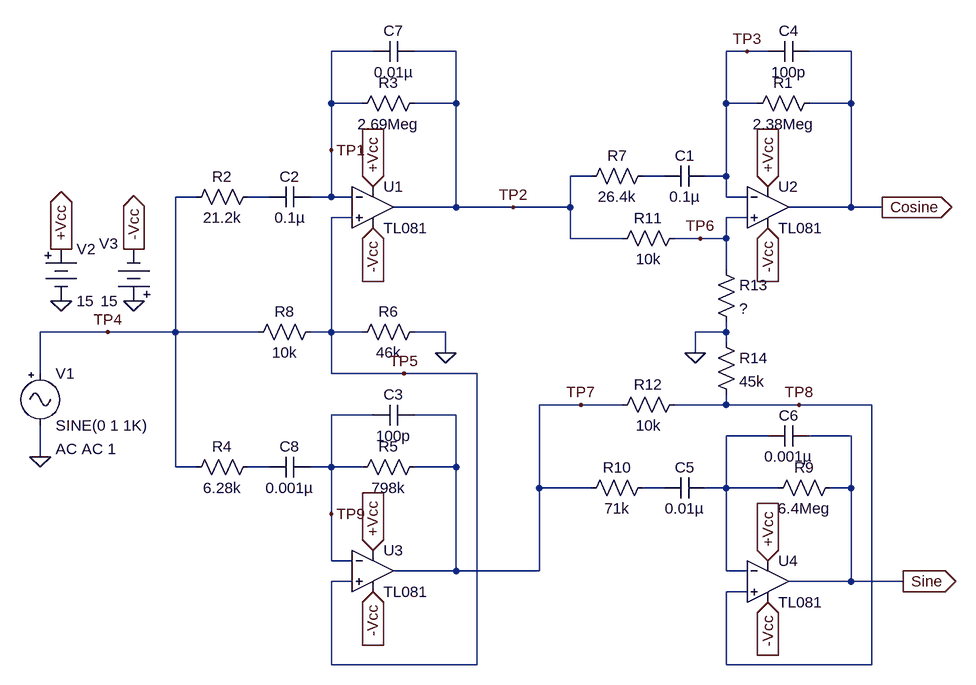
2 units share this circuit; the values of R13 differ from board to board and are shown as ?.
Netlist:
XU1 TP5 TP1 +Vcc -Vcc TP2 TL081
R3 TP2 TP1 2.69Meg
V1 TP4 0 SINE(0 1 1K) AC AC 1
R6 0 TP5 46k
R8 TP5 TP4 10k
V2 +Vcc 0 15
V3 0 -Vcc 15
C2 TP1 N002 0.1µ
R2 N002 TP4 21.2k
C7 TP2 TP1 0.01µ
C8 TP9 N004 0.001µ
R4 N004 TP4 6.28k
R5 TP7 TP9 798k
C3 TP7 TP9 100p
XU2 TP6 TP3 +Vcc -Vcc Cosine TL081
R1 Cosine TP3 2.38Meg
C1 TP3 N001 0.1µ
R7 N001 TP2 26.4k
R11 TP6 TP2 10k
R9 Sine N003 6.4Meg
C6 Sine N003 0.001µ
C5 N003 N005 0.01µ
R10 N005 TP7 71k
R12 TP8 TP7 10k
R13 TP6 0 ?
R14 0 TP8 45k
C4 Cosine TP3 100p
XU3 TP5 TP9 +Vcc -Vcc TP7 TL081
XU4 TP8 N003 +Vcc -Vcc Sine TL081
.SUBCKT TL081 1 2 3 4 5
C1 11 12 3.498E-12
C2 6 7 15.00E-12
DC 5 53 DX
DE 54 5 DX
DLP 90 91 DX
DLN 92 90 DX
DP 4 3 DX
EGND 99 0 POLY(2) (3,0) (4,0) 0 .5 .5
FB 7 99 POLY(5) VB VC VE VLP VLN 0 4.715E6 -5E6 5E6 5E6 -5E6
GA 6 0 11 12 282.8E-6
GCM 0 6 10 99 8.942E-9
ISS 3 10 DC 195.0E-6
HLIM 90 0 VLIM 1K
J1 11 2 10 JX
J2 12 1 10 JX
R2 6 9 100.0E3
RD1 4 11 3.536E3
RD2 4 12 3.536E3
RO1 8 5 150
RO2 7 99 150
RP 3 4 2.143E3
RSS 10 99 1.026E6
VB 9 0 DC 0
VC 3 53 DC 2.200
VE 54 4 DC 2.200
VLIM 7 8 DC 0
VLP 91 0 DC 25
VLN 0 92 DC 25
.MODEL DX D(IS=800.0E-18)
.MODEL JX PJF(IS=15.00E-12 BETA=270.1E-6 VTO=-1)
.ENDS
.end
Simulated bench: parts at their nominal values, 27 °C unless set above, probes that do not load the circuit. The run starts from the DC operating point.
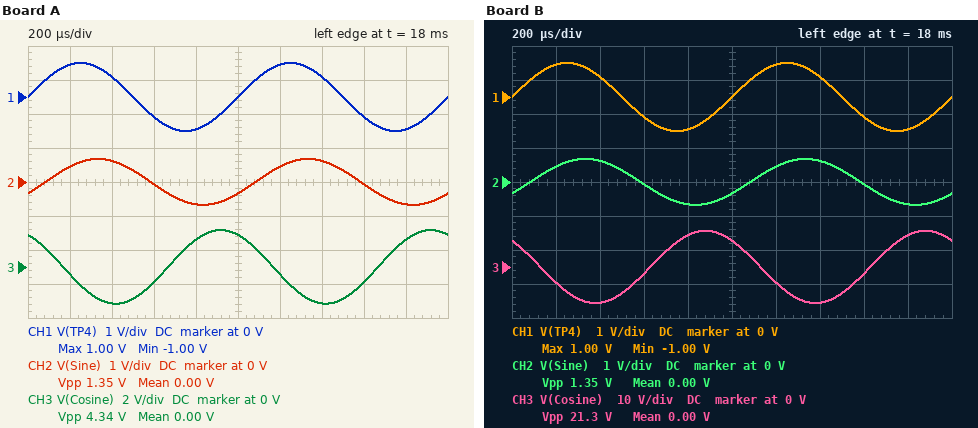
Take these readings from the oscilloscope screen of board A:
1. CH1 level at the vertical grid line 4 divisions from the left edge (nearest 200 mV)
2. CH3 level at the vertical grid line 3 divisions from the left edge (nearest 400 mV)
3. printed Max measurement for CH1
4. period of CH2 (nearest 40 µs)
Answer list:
-1.0 V
-800 mV
1.00 V
1.00 ms
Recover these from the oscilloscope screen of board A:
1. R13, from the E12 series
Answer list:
150 kΩ
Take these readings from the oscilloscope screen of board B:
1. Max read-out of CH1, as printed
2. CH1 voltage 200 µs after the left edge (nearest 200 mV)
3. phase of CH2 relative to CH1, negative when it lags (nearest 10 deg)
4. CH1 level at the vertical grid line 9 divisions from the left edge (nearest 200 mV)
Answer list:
1.00 V
1.0 V
-30 deg
-1.0 V
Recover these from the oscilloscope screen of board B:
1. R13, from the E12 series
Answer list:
27 kΩ
